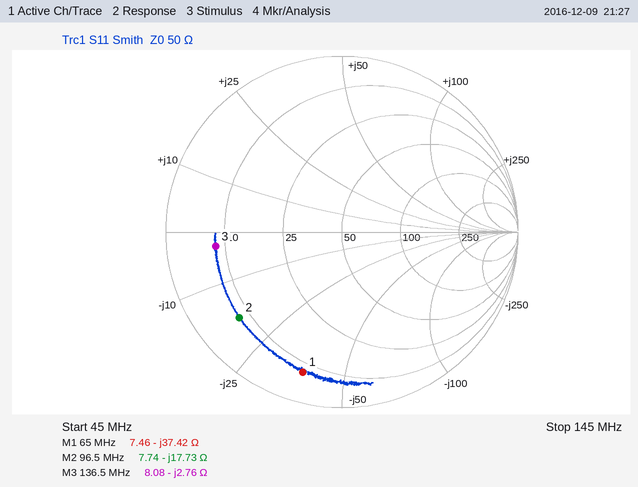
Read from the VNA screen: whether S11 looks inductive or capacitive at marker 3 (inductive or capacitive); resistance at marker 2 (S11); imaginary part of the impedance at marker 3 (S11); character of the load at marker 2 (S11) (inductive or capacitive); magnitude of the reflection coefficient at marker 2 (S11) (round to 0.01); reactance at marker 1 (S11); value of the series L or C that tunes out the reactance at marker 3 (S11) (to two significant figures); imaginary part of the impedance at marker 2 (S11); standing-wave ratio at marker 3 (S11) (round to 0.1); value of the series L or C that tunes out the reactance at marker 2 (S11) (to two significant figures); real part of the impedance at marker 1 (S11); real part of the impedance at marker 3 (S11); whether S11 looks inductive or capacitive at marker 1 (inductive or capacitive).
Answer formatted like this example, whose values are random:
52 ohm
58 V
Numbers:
capacitive
7.74 Ω
-2.76 Ω
capacitive
0.76
-37.42 Ω
3.2 nH
-17.73 Ω
6.2
29 nH
7.46 Ω
8.08 Ω
capacitive
